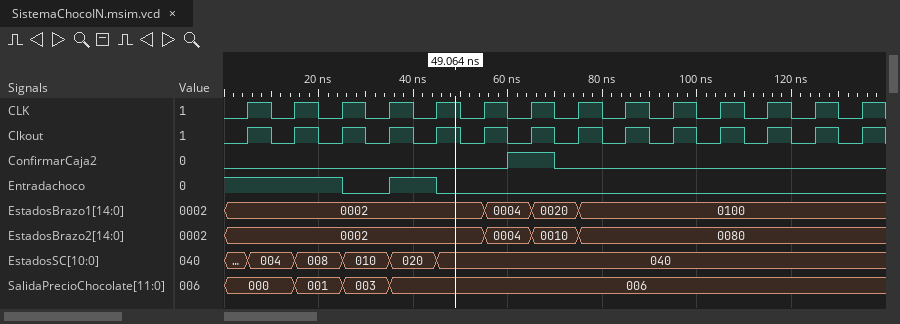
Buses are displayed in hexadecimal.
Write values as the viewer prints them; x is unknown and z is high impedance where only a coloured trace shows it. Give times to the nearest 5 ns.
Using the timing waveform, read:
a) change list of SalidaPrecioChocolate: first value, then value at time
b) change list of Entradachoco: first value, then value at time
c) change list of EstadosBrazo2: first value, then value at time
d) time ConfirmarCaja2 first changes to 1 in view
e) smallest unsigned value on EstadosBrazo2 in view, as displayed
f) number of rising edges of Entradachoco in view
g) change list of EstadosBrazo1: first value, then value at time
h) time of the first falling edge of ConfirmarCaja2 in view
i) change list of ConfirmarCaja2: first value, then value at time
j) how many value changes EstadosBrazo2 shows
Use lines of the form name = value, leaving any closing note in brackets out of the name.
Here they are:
change list of SalidaPrecioChocolate: first value, then value at time = 000, 001 at 15 ns, 003 at 25 ns, 006 at 35 ns
change list of Entradachoco: first value, then value at time = 1, 0 at 25 ns, 1 at 35 ns, 0 at 45 ns
change list of EstadosBrazo2: first value, then value at time = 0002, 0004 at 55 ns, 0010 at 65 ns, 0080 at 75 ns
time ConfirmarCaja2 first changes to 1 in view = 60 ns
smallest unsigned value on EstadosBrazo2 in view, as displayed = 0002
number of rising edges of Entradachoco in view = 1
change list of EstadosBrazo1: first value, then value at time = 0002, 0004 at 55 ns, 0020 at 65 ns, 0100 at 75 ns
time of the first falling edge of ConfirmarCaja2 in view = 70 ns
change list of ConfirmarCaja2: first value, then value at time = 0, 1 at 60 ns, 0 at 70 ns
how many value changes EstadosBrazo2 shows = 3
